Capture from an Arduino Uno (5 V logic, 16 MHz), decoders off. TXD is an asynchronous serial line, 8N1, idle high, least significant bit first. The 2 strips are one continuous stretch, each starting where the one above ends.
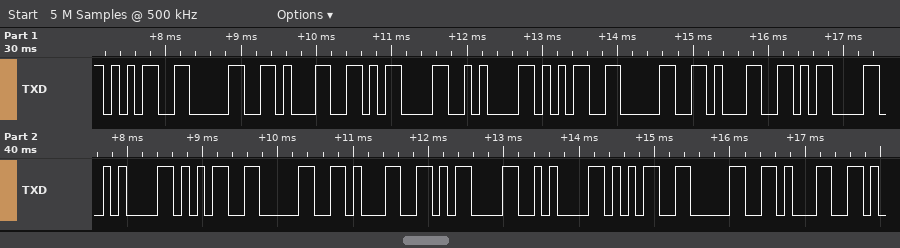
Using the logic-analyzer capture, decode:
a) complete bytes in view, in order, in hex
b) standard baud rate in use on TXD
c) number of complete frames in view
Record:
0x35 0x30 0x31 0x0D 0x0A 0x35 0x30 0x31 0x0D 0x0A 0x35 0x30 0x31 0x0D 0x0A 0x35 0x30 0x31
9600 baud
18
